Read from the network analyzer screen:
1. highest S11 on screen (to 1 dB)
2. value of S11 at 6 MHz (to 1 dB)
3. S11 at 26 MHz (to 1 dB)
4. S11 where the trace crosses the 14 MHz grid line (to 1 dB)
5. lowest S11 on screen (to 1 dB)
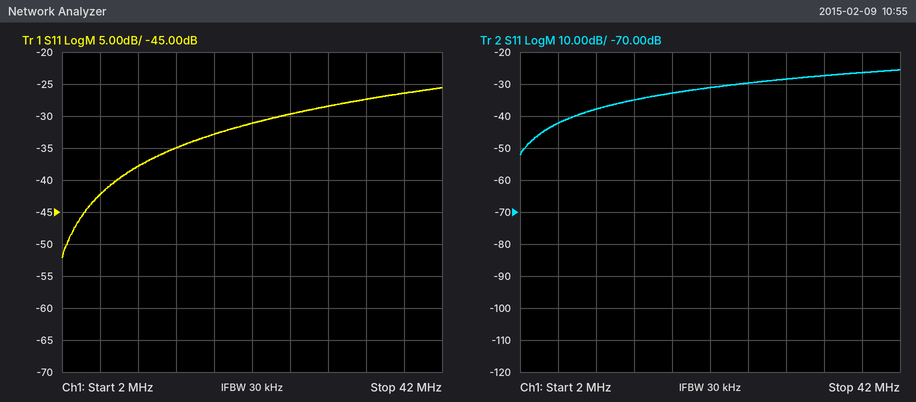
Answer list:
-26 dB
-42 dB
-30 dB
-35 dB
-52 dB
